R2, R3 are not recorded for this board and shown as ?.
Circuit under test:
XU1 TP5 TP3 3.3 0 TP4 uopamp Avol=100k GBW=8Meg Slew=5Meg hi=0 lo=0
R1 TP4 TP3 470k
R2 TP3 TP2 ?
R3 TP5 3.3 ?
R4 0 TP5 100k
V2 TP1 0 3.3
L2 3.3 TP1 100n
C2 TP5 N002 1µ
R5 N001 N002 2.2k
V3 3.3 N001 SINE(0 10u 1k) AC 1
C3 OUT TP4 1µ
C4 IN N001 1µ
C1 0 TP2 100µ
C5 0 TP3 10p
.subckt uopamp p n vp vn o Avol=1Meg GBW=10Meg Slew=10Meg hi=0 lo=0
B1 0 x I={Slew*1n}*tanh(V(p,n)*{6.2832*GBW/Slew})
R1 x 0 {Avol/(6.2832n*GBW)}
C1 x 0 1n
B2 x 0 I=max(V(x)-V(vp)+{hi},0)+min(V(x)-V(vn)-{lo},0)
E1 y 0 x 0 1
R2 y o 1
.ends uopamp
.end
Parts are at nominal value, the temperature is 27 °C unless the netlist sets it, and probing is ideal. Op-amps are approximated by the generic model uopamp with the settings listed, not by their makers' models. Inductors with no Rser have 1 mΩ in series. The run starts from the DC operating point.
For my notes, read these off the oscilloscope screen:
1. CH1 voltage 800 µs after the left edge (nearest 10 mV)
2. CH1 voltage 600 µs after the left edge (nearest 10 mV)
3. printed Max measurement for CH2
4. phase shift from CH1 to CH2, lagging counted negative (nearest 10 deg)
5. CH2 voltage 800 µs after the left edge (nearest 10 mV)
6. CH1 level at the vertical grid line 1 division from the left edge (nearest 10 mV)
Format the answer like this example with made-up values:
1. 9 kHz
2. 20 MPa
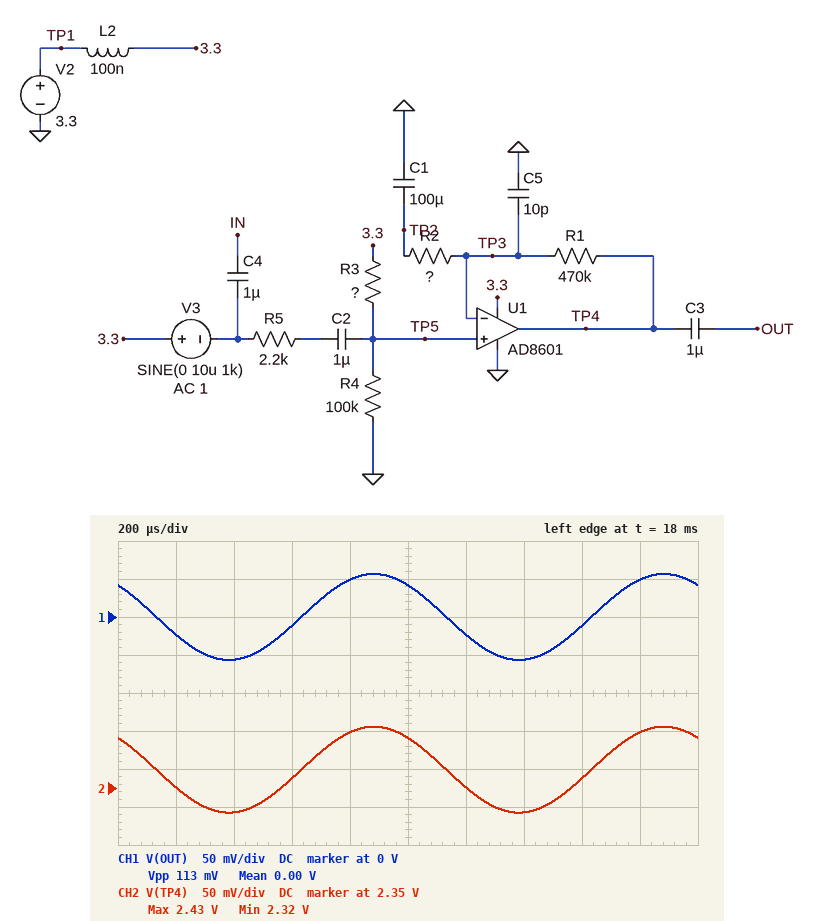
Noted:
1. 50 mV
2. -10 mV
3. 2.43 V
4. 0 deg
5. 2.42 V
6. -20 mV
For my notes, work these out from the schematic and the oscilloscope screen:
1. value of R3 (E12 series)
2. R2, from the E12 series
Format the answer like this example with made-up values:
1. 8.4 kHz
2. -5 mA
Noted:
1. 39 kΩ
2. 47 Ω
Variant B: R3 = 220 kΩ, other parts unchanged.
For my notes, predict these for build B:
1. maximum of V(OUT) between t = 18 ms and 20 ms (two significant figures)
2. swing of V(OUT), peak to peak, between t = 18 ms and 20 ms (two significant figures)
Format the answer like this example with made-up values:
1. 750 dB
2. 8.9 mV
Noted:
1. 59 mV
2. 120 mV
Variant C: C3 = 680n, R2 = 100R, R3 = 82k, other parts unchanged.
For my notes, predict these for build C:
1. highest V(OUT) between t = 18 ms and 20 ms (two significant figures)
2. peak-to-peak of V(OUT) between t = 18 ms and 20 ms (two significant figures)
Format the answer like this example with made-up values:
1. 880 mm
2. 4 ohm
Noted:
1. 38 mV
2. 75 mV
